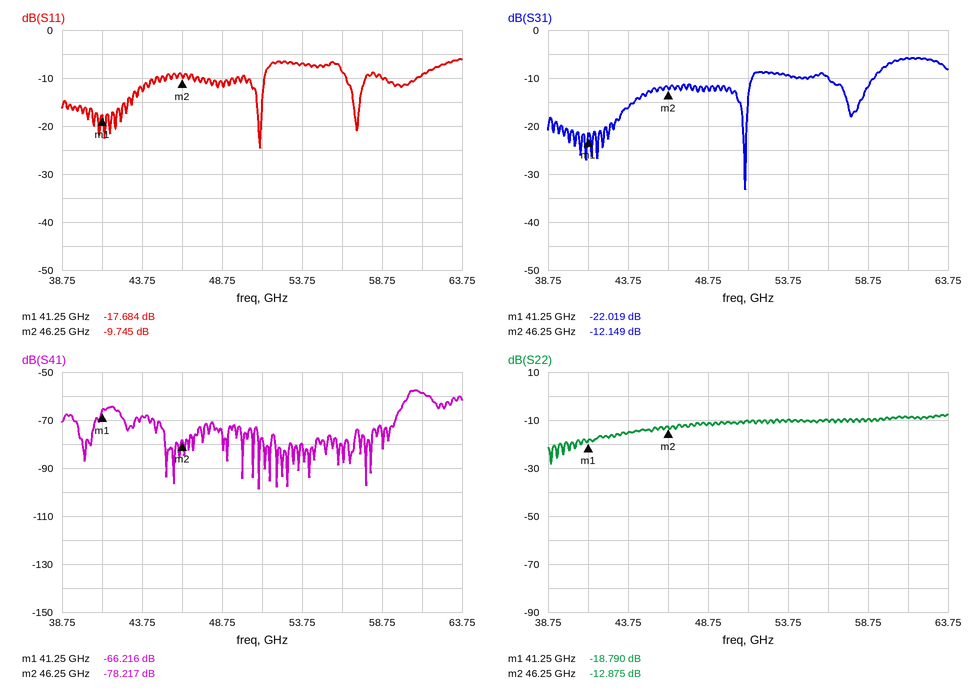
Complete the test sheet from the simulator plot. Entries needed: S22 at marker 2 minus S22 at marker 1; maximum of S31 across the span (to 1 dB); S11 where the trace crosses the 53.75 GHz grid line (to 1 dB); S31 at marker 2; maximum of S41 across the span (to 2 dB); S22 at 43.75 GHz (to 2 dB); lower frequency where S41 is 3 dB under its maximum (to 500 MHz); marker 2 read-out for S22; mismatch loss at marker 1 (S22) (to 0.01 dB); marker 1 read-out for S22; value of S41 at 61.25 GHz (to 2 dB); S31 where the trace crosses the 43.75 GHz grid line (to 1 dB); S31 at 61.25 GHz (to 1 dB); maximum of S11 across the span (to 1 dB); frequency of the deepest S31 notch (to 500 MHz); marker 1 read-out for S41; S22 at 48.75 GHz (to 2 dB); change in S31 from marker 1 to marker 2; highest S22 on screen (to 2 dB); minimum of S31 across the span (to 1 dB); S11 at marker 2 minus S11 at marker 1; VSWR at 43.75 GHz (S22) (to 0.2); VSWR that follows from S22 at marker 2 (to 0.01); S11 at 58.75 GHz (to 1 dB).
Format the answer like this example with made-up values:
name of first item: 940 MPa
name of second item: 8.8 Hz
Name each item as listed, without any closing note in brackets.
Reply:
S22 at marker 2 minus S22 at marker 1: 5.915 dB
maximum of S31 across the span: -6 dB
S11 where the trace crosses the 53.75 GHz grid line: -7 dB
S31 at marker 2: -12.149 dB
maximum of S41 across the span: -58 dB
S22 at 43.75 GHz: -16 dB
lower frequency where S41 is 3 dB under its maximum: 60.5 GHz
marker 2 read-out for S22: -12.875 dB
mismatch loss at marker 1 (S22): 0.06 dB
marker 1 read-out for S22: -18.790 dB
value of S41 at 61.25 GHz: -58 dB
S31 where the trace crosses the 43.75 GHz grid line: -16 dB
S31 at 61.25 GHz: -6 dB
maximum of S11 across the span: -6 dB
frequency of the deepest S31 notch: 51.0 GHz
marker 1 read-out for S41: -66.216 dB
S22 at 48.75 GHz: -12 dB
change in S31 from marker 1 to marker 2: 9.870 dB
highest S22 on screen: -8 dB
minimum of S31 across the span: -33 dB
S11 at marker 2 minus S11 at marker 1: 7.939 dB
VSWR at 43.75 GHz (S22): 1.4
VSWR that follows from S22 at marker 2: 1.59
S11 at 58.75 GHz: -10 dB
